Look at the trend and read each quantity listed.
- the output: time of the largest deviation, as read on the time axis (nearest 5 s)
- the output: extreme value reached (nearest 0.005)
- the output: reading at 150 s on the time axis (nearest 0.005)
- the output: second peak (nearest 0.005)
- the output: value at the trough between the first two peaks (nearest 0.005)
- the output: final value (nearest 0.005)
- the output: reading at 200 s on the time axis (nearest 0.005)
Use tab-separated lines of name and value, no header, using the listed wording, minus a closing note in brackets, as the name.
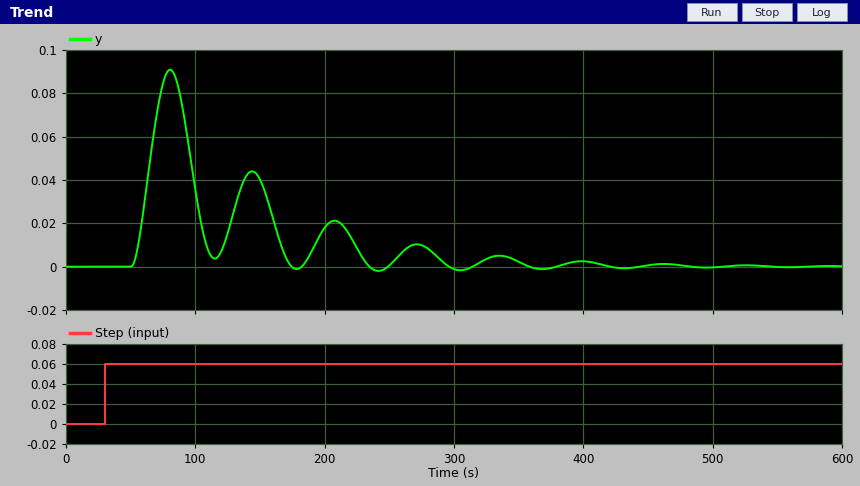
the output: time of the largest deviation, as read on the time axis	80 s
the output: extreme value reached	0.090
the output: reading at 150 s on the time axis	0.040
the output: second peak	0.045
the output: value at the trough between the first two peaks	0.005
the output: final value	0.000
the output: reading at 200 s on the time axis	0.020
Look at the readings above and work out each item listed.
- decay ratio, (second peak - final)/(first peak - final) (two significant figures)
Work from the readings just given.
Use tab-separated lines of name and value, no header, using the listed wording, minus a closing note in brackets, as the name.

decay ratio, (second peak - final)/(first peak - final)	0.50
